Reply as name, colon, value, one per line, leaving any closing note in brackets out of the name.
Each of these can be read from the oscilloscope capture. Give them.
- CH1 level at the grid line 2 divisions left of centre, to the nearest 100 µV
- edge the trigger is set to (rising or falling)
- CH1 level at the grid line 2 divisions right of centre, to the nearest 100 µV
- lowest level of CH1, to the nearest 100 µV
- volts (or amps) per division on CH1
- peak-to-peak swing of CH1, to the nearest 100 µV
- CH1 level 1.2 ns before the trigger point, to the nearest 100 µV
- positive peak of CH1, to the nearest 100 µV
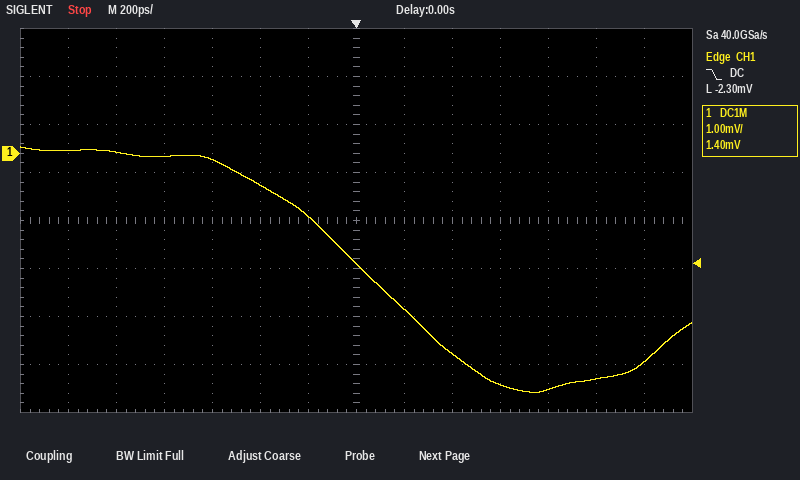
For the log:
CH1 level at the grid line 2 divisions left of centre, to the nearest 100 µV: -700 µV
edge the trigger is set to: falling
CH1 level at the grid line 2 divisions right of centre, to the nearest 100 µV: -4.2 mV
lowest level of CH1, to the nearest 100 µV: -5.0 mV
volts (or amps) per division on CH1: 1 mV
peak-to-peak swing of CH1, to the nearest 100 µV: 5.1 mV
CH1 level 1.2 ns before the trigger point, to the nearest 100 µV: 100 µV
positive peak of CH1, to the nearest 100 µV: 100 µV
